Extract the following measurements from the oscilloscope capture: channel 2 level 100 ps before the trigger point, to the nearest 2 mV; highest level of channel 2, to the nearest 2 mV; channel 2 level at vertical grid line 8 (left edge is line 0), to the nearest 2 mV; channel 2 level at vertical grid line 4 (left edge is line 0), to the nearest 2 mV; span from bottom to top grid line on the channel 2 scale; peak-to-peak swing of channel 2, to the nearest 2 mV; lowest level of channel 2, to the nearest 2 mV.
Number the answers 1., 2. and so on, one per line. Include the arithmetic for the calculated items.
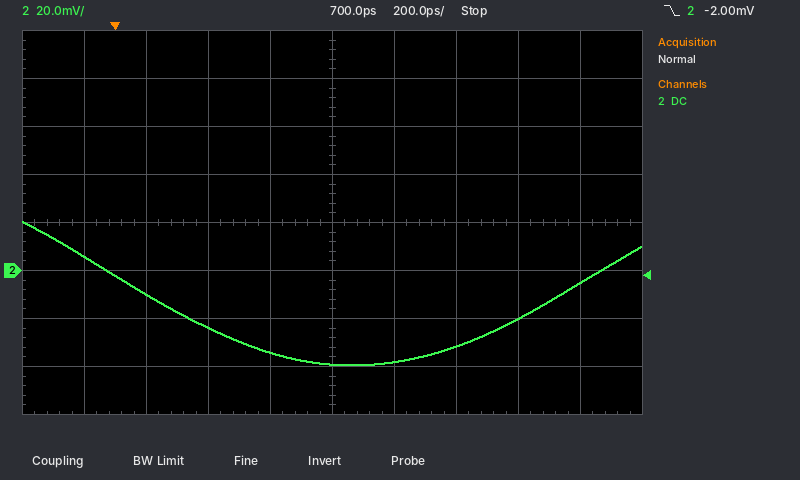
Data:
1. 6 mV
2. 20 mV
3. -20 mV
4. -34 mV
5. 160 mV
6. 20 mV − (-40 mV) = 60 mV
7. -40 mV
